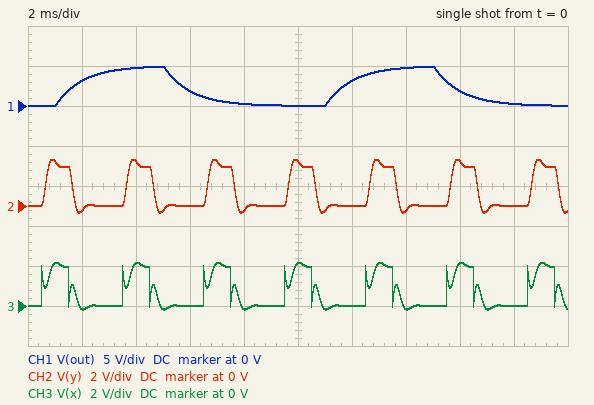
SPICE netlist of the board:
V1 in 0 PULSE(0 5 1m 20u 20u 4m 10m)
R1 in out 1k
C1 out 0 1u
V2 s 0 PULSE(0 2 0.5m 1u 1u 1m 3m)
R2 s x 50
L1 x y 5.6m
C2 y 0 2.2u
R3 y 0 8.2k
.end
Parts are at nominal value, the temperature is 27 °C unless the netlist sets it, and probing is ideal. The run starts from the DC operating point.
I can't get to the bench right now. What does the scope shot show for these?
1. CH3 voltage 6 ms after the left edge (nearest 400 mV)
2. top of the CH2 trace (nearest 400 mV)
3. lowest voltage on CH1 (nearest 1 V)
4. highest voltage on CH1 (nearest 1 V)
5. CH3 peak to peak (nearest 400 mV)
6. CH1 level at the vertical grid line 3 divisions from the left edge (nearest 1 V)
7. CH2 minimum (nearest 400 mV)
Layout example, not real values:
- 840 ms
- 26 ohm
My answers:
- 0 V
- 2.4 V
- 0 V
- 5 V
- 2.4 V
- 2 V
- -400 mV
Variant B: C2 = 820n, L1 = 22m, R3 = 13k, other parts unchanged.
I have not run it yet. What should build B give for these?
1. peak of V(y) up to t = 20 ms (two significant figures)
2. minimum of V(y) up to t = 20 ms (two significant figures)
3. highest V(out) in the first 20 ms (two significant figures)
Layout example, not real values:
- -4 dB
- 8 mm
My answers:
- 3.2 V
- -1.0 V
- 4.9 V
